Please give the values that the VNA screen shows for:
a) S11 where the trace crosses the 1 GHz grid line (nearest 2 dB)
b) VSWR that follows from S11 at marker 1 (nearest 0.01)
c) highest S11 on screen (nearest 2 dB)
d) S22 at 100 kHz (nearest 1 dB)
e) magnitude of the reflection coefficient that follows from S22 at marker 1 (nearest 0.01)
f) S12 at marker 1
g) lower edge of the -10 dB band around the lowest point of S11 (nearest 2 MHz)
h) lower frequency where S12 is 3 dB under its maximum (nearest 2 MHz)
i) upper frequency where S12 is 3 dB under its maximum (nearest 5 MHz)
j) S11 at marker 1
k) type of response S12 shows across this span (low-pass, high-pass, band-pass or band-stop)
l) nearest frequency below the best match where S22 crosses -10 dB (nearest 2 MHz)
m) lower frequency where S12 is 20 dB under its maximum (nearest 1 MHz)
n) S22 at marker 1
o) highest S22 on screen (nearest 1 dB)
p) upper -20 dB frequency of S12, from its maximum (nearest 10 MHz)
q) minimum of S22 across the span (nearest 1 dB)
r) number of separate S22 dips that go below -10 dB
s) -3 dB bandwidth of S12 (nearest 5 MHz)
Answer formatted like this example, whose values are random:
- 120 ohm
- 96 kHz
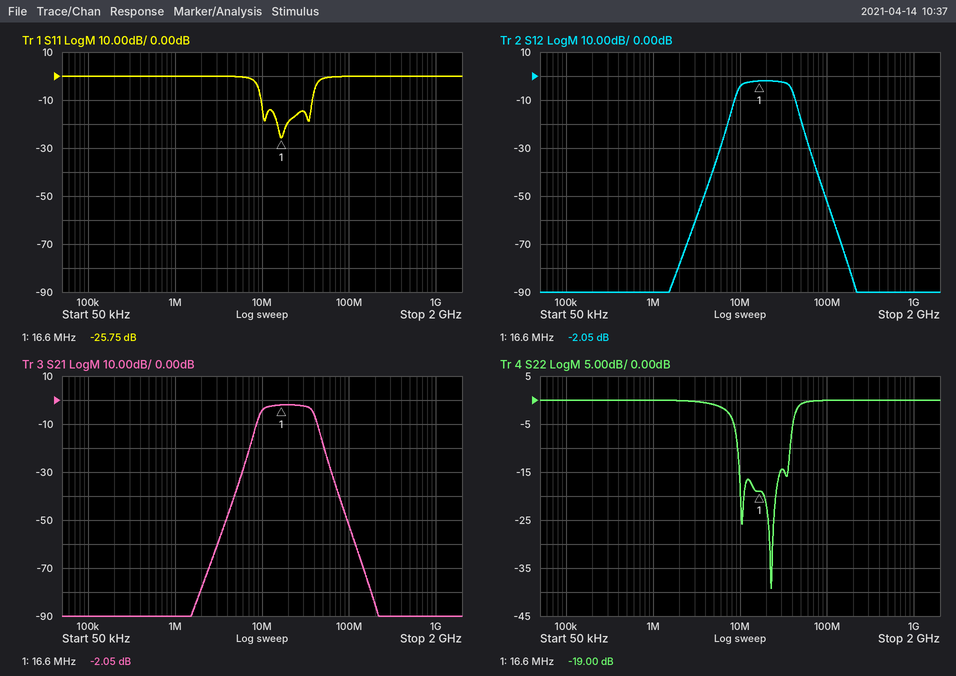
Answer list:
- 0 dB
- 1.11
- 0 dB
- 0 dB
- 0.11
- -2.05 dB
- 10 MHz
- 10 MHz
- 40 MHz
- -25.75 dB
- band-pass
- 10 MHz
- 7 MHz
- -19.00 dB
- 0 dB
- 50 MHz
- -39 dB
- 2
- 30 MHz
